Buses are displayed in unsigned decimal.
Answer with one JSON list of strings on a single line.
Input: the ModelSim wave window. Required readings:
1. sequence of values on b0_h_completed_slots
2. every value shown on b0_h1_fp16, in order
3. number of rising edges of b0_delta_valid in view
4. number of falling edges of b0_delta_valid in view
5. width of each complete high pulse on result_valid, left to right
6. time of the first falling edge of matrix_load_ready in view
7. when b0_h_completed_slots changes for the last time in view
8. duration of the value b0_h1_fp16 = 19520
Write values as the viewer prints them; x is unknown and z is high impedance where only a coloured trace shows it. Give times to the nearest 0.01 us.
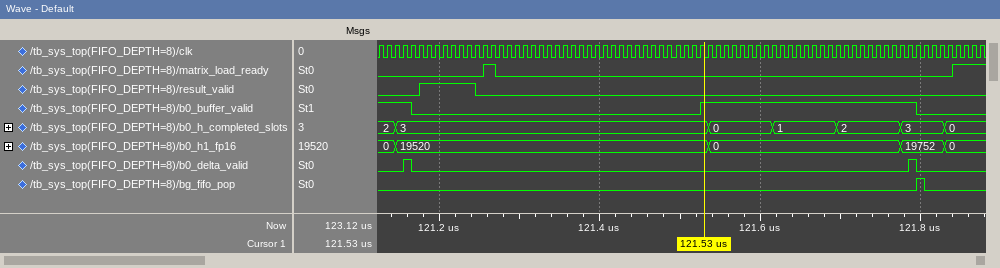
["2, 3, 0, 1, 2, 3, 0", "0, 19520, 0, 19752, 0", "2", "2", "0.07 us", "121.27 us", "121.83 us", "0.39 us"]
